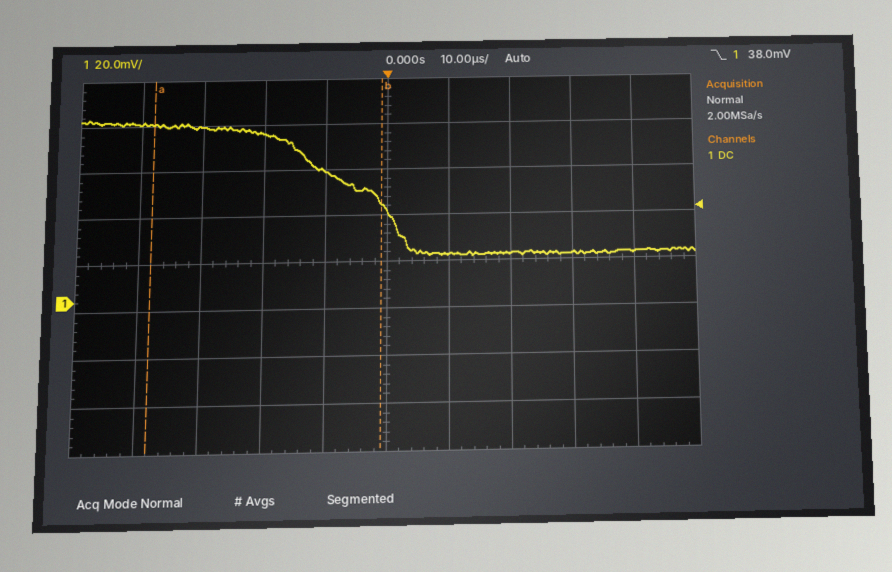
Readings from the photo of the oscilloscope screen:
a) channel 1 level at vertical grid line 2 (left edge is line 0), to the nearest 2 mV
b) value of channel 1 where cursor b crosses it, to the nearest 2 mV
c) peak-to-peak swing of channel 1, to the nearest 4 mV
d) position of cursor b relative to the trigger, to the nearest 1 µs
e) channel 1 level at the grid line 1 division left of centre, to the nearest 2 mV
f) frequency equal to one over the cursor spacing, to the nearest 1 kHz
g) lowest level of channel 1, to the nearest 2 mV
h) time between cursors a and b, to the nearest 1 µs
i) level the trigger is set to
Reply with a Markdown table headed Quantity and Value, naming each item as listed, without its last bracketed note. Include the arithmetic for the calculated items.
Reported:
| Quantity | Value |
|---|---|
| channel 1 level at vertical grid line 2 (left edge is line 0), to the nearest 2 mV | 76 mV |
| value of channel 1 where cursor b crosses it, to the nearest 2 mV | 42 mV |
| peak-to-peak swing of channel 1, to the nearest 4 mV | 60 mV |
| position of cursor b relative to the trigger, to the nearest 1 µs | -1 µs |
| channel 1 level at the grid line 1 division left of centre, to the nearest 2 mV | 56 mV |
| frequency equal to one over the cursor spacing, to the nearest 1 kHz | 1 / 37 µs ≈ 27 kHz |
| lowest level of channel 1, to the nearest 2 mV | 18 mV |
| time between cursors a and b, to the nearest 1 µs | 37 µs |
| level the trigger is set to | 38.0 mV |
